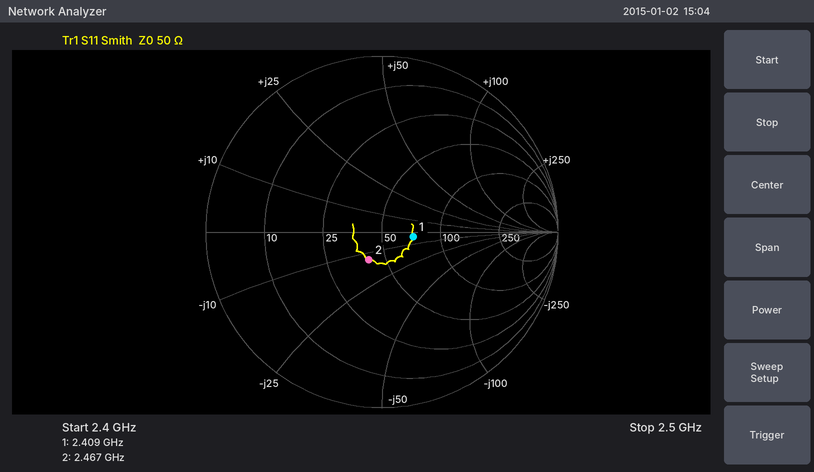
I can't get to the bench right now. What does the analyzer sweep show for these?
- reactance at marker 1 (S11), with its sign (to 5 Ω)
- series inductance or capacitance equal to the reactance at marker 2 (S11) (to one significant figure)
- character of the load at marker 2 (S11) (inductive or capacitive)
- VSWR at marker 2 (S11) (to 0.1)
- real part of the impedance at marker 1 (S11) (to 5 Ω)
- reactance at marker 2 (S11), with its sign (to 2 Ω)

-5 Ω
5 pF
capacitive
1.4
70 Ω
-14 Ω
